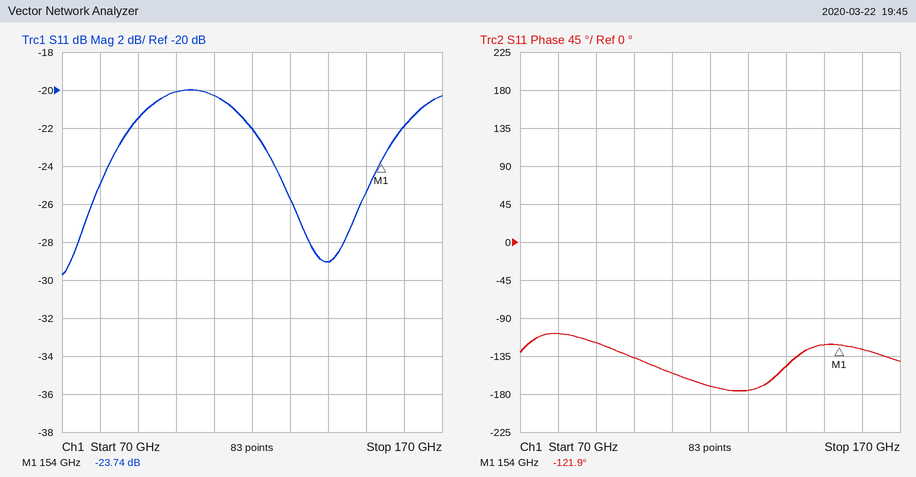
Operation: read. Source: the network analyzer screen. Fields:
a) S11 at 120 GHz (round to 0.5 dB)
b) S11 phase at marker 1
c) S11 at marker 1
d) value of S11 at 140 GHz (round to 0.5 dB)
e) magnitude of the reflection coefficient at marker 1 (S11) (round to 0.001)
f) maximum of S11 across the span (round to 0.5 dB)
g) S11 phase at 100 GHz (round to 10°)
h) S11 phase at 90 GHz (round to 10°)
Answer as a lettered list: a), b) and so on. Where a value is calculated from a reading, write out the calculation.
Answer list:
a) -22.0 dB
b) -121.9°
c) -23.74 dB
d) -29.0 dB
e) 10^(-23.74/20) ≈ 0.065
f) -20.0 dB
g) -140°
h) -120°
